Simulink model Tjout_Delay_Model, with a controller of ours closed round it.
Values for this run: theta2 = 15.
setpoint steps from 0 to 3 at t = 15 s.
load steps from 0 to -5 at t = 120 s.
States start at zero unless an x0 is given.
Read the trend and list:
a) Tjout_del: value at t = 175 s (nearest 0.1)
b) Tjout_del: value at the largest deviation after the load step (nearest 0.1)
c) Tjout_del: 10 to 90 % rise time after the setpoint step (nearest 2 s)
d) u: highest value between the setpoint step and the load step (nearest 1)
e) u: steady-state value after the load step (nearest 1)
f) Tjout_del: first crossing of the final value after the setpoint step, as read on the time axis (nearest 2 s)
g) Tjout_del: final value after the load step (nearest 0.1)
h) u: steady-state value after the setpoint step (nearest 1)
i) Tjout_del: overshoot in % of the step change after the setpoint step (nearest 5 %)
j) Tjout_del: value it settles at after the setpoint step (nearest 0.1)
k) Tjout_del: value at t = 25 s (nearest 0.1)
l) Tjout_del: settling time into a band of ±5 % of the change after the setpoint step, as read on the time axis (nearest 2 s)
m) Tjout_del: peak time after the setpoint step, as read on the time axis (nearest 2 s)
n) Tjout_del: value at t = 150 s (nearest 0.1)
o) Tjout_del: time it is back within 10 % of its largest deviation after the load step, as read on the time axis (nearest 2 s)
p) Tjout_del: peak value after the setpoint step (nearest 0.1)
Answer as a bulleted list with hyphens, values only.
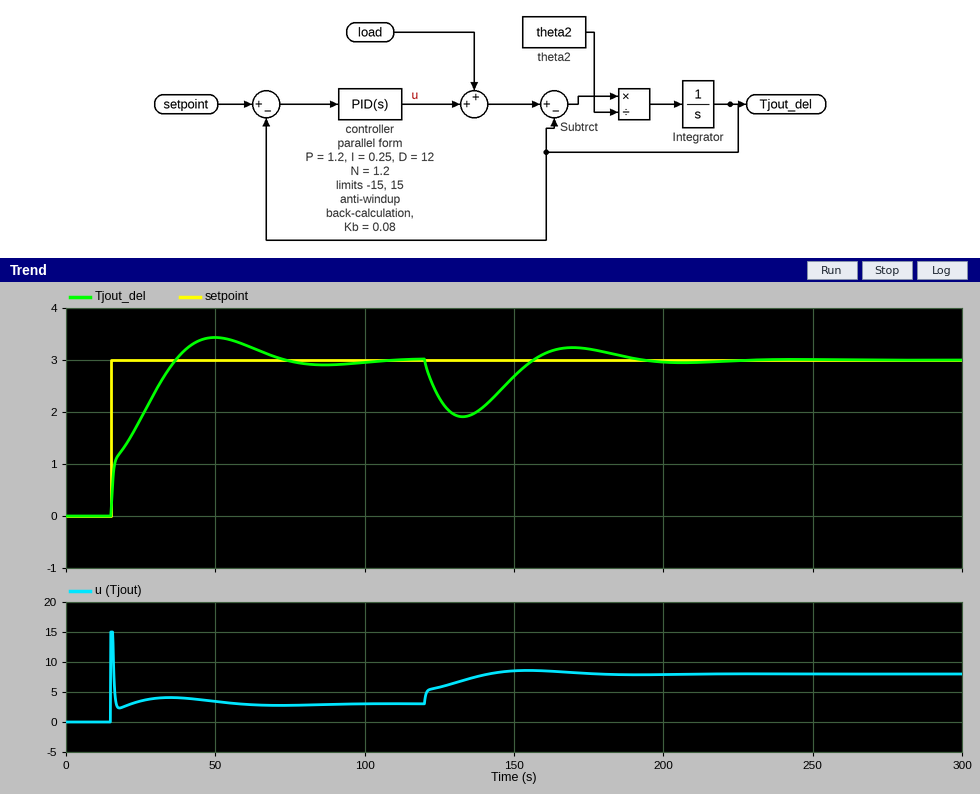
- 3.2
- 1.9
- 18 s
- 15
- 8
- 36 s
- 3.0
- 3
- 15 %
- 3.0
- 1.9
- 66 s
- 50 s
- 2.7
- 184 s
- 3.4
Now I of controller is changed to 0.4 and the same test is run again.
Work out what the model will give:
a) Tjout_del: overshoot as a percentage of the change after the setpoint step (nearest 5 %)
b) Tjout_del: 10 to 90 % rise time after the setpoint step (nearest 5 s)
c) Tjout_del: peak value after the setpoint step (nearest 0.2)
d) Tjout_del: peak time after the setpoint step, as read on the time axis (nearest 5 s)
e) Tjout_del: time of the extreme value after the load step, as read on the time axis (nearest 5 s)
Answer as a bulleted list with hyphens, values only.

- 20 %
- 15 s
- 3.6
- 40 s
- 130 s
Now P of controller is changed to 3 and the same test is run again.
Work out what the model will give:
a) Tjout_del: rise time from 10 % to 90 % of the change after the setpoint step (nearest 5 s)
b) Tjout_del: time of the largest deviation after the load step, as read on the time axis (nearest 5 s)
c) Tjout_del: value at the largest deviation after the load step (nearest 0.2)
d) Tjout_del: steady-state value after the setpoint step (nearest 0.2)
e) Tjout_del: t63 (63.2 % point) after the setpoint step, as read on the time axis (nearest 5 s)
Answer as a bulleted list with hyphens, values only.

- 15 s
- 130 s
- 2.2
- 3.0
- 20 s
